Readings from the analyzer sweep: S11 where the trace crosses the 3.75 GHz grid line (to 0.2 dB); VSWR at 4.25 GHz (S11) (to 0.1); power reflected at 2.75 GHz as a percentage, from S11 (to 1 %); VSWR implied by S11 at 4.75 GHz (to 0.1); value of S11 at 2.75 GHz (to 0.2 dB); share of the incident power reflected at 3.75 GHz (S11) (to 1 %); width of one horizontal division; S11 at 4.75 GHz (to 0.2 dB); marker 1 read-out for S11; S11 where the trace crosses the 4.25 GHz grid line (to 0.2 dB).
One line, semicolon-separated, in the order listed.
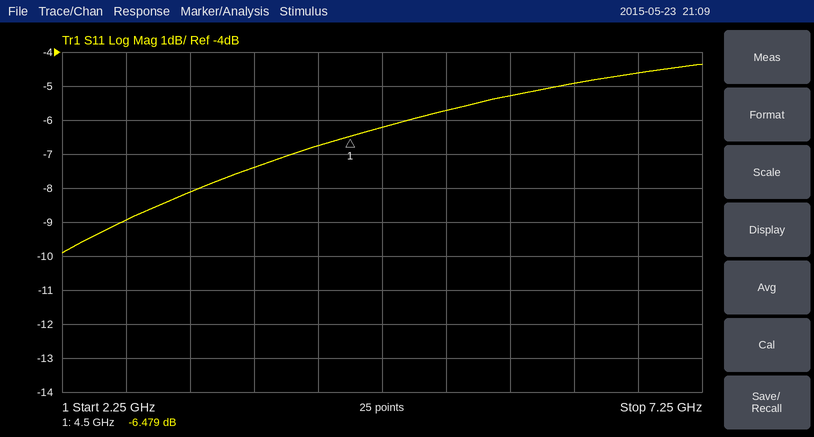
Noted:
-7.4 dB; 2.7; 13 %; 2.9; -9.0 dB; 18 %; 500 MHz; -6.2 dB; -6.479 dB; -6.8 dB
